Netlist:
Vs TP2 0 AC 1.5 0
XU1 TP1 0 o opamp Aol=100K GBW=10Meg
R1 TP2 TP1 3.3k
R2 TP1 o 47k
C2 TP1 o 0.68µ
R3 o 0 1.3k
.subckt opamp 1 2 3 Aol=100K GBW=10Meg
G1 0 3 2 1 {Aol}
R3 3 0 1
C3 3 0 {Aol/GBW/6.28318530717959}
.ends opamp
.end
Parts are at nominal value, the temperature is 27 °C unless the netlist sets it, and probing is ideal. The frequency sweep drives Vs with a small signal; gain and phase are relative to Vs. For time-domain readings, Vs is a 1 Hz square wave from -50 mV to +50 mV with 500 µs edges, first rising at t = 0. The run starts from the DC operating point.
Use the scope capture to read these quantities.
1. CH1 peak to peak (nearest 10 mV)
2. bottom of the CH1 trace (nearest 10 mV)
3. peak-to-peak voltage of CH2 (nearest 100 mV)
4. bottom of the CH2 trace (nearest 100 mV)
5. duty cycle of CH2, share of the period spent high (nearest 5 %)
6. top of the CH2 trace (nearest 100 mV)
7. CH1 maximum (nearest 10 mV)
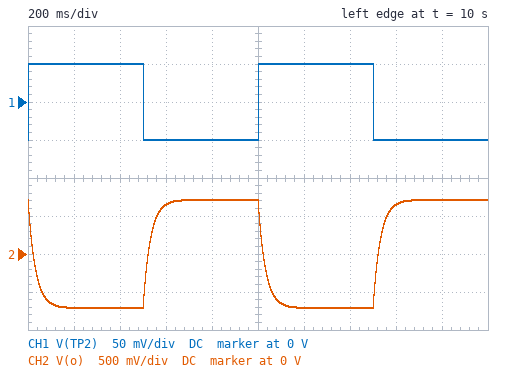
100 mV
-50 mV
1.4 V
-700 mV
50 %
700 mV
50 mV
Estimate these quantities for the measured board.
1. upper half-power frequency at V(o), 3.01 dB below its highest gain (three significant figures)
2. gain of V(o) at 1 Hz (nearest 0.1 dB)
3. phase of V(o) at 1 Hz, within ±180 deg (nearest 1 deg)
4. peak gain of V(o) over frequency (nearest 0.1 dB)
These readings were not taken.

4.98 Hz
22.9 dB
169 deg
23.1 dB
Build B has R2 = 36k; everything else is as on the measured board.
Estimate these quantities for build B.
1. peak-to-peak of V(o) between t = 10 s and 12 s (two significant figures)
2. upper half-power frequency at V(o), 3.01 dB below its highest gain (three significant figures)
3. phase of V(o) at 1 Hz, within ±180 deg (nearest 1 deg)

1.1 V
6.50 Hz
171 deg
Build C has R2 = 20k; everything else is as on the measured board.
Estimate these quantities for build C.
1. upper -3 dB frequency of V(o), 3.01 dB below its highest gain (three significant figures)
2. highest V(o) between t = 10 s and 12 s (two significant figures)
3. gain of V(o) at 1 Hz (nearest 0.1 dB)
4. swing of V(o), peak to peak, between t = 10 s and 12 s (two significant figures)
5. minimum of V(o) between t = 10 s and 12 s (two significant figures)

11.7 Hz
300 mV
15.6 dB
610 mV
-300 mV
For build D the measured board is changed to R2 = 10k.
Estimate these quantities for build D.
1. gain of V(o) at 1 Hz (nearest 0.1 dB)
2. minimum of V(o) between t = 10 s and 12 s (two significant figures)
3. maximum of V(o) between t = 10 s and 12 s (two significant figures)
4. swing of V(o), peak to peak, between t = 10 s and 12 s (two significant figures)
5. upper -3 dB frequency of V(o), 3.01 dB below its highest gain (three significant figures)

9.6 dB
-150 mV
150 mV
300 mV
23.4 Hz
